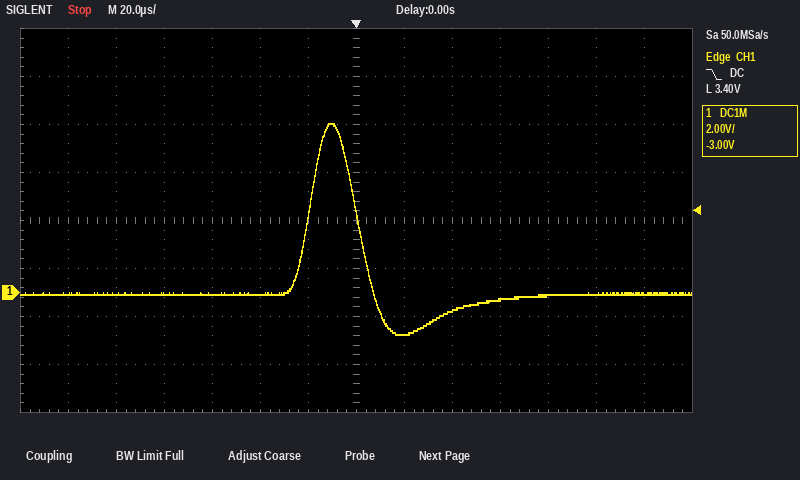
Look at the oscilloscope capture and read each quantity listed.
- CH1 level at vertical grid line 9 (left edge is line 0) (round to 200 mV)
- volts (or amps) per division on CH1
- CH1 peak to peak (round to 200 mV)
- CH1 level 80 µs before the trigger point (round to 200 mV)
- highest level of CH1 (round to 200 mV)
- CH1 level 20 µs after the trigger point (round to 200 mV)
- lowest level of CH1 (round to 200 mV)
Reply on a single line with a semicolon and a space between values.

-800 mV; 2 V; 8.8 V; 0.0 V; 7.0 V; -1.8 V; -1.8 V
